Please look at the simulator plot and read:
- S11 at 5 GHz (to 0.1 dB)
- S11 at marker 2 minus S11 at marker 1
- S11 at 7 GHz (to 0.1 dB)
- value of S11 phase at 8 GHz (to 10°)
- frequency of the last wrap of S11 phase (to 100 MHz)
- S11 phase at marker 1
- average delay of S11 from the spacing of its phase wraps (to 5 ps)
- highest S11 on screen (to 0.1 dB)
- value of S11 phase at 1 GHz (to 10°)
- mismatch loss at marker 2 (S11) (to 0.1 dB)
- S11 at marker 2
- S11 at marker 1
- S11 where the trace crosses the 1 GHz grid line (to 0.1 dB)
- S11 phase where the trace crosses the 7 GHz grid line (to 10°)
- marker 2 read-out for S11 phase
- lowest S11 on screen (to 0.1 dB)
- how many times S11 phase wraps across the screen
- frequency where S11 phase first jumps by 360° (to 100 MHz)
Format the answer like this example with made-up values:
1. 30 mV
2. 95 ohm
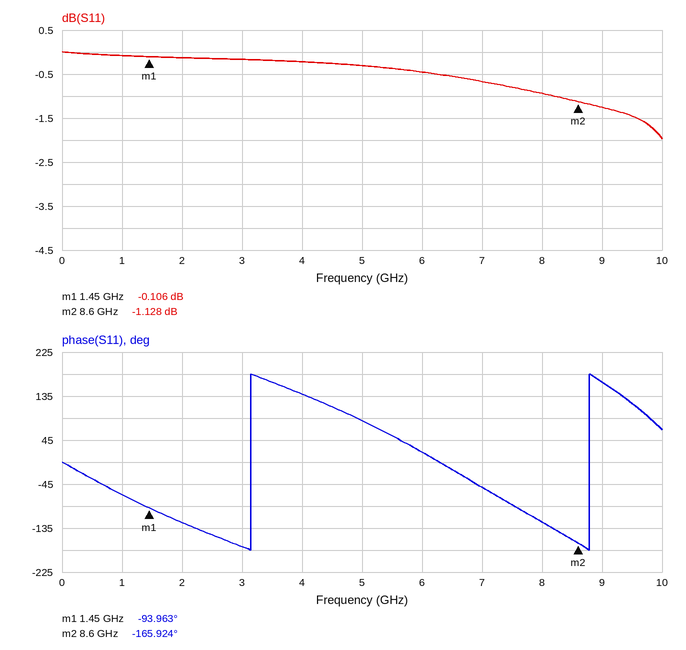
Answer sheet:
1. -0.3 dB
2. -1.022 dB
3. -0.7 dB
4. -120°
5. 8.8 GHz
6. -93.963°
7. 175 ps
8. 0.0 dB
9. -70°
10. 6.4 dB
11. -1.128 dB
12. -0.106 dB
13. -0.1 dB
14. -50°
15. -165.924°
16. -2.0 dB
17. 2
18. 3.1 GHz
